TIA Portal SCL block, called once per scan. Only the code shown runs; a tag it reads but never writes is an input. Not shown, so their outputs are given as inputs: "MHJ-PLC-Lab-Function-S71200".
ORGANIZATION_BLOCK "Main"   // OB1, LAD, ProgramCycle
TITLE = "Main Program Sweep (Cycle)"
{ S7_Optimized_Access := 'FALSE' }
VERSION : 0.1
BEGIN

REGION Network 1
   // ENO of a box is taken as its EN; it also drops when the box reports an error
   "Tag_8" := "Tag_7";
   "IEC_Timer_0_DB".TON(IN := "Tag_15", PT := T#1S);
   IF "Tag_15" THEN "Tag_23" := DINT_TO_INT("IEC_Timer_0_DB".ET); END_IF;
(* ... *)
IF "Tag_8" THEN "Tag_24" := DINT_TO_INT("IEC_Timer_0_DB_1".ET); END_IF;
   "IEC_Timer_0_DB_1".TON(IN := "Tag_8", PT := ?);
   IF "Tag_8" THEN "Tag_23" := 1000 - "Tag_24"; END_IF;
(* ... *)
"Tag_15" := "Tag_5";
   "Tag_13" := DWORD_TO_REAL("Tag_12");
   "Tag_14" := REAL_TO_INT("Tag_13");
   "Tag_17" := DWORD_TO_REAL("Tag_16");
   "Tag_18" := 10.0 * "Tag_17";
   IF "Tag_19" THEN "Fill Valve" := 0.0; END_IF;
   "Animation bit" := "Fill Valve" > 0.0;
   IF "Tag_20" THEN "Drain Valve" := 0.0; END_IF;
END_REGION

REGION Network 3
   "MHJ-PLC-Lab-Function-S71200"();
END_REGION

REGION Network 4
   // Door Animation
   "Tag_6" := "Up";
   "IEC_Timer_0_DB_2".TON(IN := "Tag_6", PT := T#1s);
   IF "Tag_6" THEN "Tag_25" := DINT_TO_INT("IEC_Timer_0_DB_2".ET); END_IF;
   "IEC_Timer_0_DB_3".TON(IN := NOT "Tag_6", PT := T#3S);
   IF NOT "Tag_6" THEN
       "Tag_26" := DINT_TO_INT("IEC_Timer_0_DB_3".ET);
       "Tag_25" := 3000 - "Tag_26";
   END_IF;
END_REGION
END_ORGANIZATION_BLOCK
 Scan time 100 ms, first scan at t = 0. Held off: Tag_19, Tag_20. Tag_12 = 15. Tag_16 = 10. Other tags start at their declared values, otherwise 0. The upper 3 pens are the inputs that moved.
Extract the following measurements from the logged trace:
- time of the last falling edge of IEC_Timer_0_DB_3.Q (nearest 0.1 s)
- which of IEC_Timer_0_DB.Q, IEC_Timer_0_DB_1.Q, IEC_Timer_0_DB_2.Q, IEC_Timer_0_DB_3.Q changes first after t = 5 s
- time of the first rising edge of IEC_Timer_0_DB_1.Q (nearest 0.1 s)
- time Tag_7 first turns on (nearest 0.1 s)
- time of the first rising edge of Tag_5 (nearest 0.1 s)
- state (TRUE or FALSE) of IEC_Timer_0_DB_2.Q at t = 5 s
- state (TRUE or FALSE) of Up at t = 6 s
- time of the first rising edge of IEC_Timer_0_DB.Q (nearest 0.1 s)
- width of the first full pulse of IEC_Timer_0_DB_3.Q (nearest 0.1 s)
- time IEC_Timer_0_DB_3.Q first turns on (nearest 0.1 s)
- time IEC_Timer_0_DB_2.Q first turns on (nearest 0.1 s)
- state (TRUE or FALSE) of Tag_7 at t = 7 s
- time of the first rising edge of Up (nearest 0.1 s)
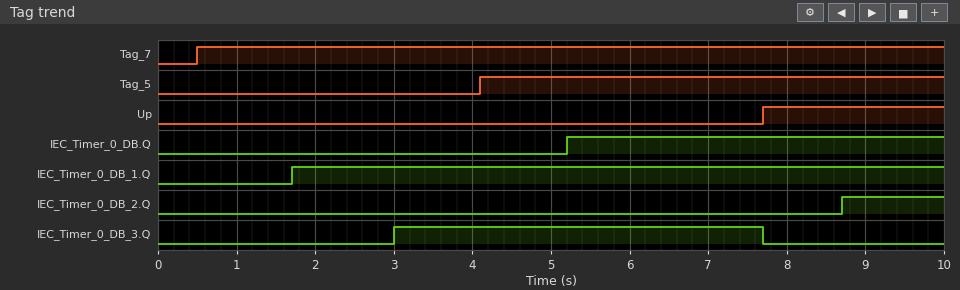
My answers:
7.7 s
IEC_Timer_0_DB.Q
1.7 s
0.5 s
4.1 s
FALSE
FALSE
5.2 s
4.7 s
3.0 s
8.7 s
TRUE
7.7 s
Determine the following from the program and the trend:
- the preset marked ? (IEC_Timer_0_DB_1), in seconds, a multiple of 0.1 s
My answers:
1.2 s
